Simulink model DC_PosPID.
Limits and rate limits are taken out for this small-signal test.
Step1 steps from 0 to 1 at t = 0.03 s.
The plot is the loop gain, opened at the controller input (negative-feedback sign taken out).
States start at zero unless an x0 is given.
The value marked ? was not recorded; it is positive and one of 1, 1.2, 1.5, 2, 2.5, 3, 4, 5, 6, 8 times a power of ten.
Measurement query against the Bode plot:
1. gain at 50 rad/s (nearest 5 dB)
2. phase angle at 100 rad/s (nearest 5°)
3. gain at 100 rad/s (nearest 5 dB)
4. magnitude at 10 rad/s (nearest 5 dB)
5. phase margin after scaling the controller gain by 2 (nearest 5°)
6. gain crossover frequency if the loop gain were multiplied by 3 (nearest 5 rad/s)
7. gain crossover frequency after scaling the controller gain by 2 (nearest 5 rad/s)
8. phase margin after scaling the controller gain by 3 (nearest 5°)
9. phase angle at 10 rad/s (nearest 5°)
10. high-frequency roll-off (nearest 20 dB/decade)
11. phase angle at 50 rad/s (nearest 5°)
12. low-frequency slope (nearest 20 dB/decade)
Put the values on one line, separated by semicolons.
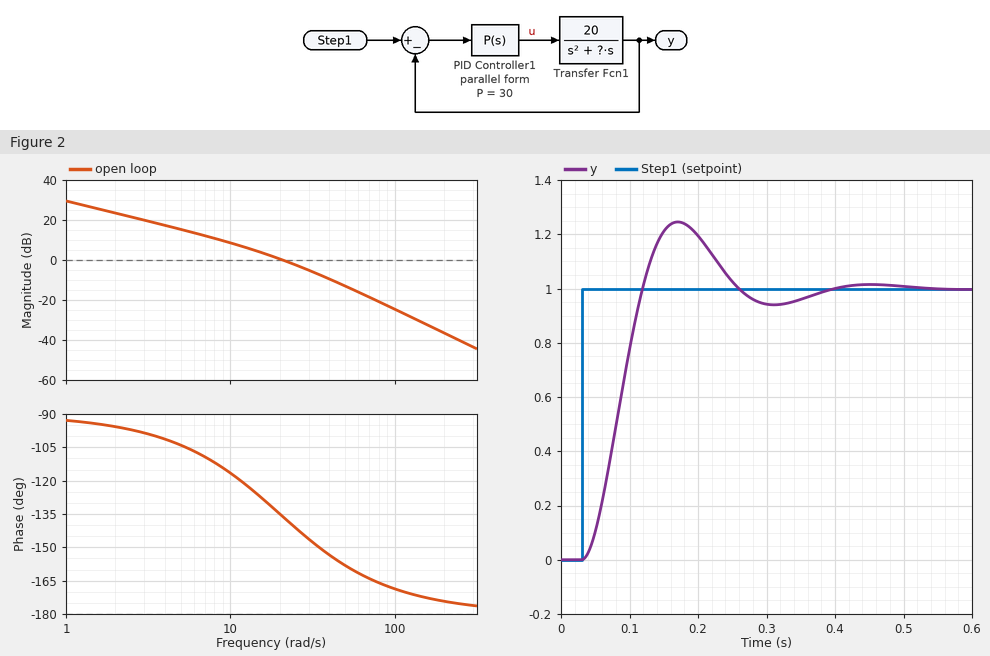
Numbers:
-15 dB; -170°; -25 dB; 10 dB; 30°; 40 rad/s; 30 rad/s; 25°; -115°; -40 dB/decade; -160°; -20 dB/decade
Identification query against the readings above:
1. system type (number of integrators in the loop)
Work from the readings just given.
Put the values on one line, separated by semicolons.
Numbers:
1
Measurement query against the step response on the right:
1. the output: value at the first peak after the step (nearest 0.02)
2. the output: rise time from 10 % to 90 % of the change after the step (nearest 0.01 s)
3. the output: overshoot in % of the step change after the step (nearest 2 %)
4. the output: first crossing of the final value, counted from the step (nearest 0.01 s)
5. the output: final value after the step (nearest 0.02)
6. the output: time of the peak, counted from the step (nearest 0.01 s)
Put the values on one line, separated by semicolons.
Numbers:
1.24; 0.06 s; 24 %; 0.09 s; 1.00; 0.14 s
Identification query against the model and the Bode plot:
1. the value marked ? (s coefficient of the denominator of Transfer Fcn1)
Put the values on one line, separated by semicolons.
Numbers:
20
